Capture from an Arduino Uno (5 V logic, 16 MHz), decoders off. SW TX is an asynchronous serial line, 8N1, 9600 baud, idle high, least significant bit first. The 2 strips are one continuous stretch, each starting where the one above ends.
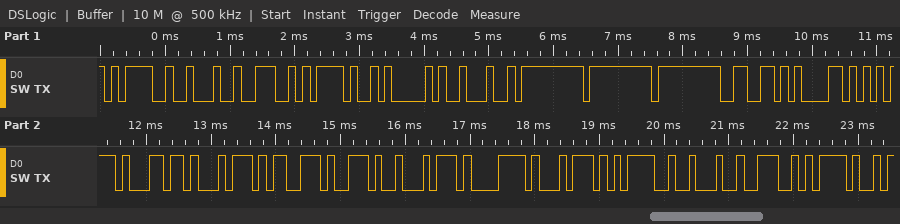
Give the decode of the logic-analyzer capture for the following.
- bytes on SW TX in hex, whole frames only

0x3D 0x22 0x4E 0x2F 0x41 0x22 0xFF 0xFF 0xFF 0x66 0x61 0x75 0x6C 0x74 0x73 0x2E 0x74 0x78 0x74 0x3D 0x22 0x4E 0x2F
